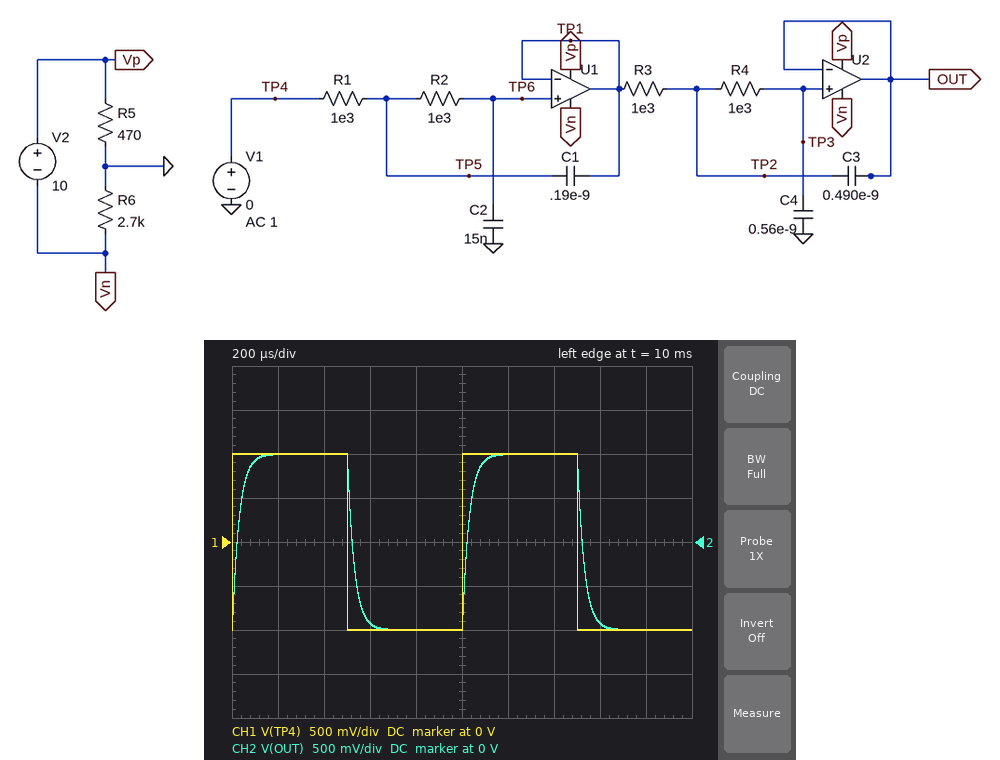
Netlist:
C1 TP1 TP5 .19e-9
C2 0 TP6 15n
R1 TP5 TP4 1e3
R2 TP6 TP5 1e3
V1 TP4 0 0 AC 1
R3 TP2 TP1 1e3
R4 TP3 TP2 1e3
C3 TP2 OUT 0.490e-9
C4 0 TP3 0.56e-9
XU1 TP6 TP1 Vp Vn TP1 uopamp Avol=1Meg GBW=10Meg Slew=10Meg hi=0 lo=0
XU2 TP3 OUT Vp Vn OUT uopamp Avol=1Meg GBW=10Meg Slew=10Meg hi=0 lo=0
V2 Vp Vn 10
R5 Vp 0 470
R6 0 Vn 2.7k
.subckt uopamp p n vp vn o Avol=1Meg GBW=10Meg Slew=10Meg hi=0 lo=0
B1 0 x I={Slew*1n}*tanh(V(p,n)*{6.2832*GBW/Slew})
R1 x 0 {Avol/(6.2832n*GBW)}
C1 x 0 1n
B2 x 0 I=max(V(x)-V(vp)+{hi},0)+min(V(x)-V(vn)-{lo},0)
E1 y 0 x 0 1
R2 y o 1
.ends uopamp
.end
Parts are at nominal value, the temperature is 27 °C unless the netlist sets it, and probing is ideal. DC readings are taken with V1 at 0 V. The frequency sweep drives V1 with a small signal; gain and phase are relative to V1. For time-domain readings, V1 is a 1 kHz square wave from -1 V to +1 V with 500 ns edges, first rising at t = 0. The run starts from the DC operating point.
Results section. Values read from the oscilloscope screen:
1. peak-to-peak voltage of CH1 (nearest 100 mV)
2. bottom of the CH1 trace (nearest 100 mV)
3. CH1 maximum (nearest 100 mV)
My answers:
2.0 V
-1.0 V
1.0 V
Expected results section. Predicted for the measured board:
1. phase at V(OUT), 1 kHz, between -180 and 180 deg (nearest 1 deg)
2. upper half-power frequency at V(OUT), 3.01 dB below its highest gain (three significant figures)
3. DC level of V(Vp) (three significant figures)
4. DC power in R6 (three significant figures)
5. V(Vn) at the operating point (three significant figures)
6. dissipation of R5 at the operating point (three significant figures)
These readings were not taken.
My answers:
-11 deg
5.32 kHz
1.48 V
26.9 mW
-8.52 V
4.68 mW
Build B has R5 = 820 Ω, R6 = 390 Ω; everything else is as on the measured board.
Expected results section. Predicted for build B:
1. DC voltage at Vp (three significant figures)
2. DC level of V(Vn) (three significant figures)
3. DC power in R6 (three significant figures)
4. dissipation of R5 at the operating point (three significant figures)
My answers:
6.78 V
-3.22 V
26.6 mW
56.0 mW
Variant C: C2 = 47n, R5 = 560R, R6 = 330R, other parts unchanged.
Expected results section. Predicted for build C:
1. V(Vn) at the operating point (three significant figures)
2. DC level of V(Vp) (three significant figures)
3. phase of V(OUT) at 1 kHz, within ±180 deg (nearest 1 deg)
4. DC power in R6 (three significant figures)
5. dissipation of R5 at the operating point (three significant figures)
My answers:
-3.71 V
6.29 V
-31 deg
41.7 mW
70.7 mW
